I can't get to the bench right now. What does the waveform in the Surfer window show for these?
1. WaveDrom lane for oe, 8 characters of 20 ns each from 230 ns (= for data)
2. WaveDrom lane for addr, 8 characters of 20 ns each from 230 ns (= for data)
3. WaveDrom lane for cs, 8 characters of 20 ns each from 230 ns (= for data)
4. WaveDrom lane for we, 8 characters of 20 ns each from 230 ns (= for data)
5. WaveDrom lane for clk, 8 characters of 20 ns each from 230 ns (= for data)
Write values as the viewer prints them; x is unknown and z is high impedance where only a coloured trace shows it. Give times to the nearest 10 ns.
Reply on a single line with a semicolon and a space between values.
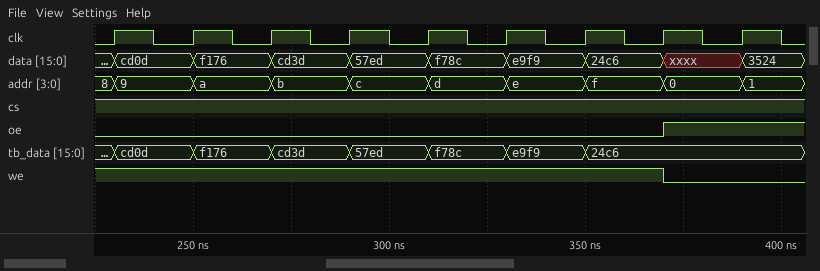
{name: 'oe', wave: '0......1'}; {name: 'addr', wave: '========', data: '9 a b c d e f 0'}; {name: 'cs', wave: '1.......'}; {name: 'we', wave: '1......0'}; {name: 'clk', wave: 'p.......'}
